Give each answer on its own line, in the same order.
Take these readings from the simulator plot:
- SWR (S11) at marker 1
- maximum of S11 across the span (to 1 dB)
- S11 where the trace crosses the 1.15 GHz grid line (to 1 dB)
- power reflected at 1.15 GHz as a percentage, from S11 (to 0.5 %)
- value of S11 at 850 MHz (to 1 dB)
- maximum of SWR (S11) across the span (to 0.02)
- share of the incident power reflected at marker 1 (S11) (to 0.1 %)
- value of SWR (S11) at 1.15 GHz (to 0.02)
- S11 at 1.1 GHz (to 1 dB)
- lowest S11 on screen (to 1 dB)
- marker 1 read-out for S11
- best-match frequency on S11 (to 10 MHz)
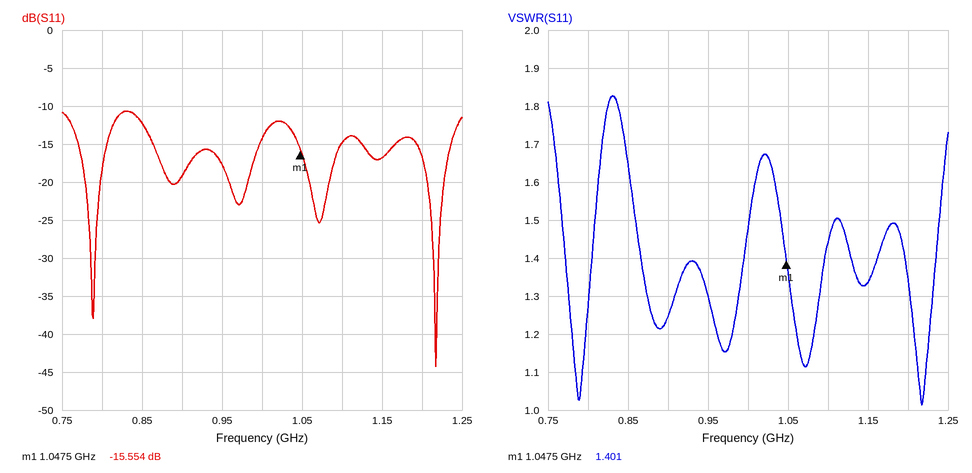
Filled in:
1.401
-11 dB
-17 dB
2.0 %
-12 dB
1.82
2.8 %
1.34
-15 dB
-44 dB
-15.554 dB
1.22 GHz
